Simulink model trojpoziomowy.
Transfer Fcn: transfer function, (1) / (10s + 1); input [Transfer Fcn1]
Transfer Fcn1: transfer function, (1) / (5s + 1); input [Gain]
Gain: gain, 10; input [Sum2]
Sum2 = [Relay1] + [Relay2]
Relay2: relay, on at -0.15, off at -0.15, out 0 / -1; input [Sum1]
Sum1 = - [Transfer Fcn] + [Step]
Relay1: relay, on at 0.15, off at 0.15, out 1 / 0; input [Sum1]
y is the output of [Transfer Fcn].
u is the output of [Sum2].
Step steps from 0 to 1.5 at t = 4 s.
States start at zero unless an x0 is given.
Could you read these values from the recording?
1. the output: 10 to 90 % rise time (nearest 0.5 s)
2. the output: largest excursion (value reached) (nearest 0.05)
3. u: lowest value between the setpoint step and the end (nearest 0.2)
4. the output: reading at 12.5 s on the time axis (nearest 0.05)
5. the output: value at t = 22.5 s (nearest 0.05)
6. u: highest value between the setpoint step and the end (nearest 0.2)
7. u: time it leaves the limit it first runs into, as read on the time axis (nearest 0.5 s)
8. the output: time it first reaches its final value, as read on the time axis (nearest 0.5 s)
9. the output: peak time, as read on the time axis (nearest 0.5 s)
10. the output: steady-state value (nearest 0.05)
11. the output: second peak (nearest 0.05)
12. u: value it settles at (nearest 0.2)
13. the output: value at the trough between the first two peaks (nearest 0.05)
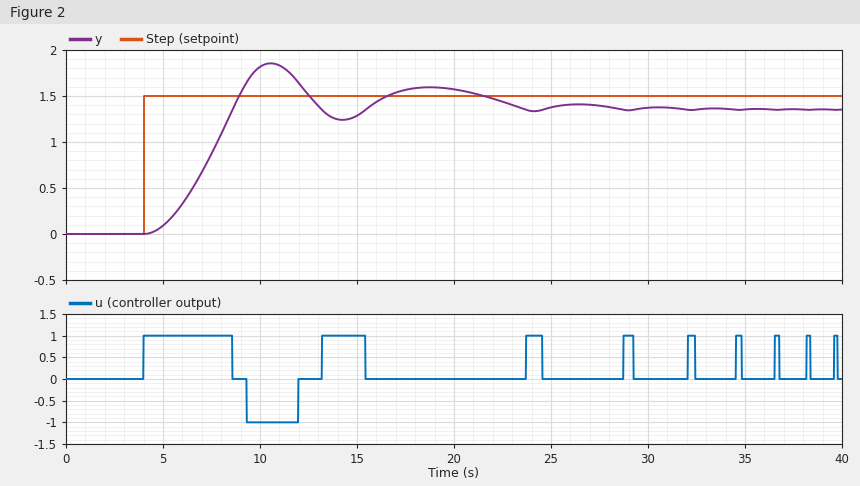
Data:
3.0 s
1.85
-1.0
1.50
1.45
1.0
8.5 s
8.5 s
10.5 s
1.35
1.60
0.0
1.25
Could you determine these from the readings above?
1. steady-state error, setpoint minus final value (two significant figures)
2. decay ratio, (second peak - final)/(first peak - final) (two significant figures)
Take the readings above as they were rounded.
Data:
0.15
0.50
